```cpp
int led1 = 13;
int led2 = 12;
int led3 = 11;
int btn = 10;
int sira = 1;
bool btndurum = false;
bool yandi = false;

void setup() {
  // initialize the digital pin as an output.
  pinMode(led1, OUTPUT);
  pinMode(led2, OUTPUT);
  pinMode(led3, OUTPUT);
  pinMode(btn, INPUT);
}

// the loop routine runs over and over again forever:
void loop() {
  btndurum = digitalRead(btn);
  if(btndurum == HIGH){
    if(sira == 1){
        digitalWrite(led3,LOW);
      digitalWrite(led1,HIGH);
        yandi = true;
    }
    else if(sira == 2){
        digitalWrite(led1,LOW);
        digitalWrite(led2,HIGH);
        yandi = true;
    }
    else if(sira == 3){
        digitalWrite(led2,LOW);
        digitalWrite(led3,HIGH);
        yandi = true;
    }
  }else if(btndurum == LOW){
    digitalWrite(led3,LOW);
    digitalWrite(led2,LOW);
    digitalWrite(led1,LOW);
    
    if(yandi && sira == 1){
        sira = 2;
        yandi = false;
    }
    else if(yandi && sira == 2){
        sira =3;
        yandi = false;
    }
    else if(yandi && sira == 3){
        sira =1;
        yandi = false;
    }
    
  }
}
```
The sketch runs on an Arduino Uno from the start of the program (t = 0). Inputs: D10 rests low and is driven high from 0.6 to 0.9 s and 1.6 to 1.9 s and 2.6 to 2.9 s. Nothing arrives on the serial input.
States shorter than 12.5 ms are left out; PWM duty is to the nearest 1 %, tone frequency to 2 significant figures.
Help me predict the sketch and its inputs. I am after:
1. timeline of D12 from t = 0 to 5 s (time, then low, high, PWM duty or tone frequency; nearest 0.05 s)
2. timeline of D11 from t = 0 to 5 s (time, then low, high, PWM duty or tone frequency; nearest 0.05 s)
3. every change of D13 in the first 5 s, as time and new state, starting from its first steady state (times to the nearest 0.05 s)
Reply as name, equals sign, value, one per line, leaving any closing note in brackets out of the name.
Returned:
timeline of D12 from t = 0 to 5 s = 0 s low; 1.6 s high; 1.9 s low
timeline of D11 from t = 0 to 5 s = 0 s low; 2.6 s high; 2.9 s low
every change of D13 in the first 5 s, as time and new state, starting from its first steady state = 0 s low; 0.6 s high; 0.9 s low
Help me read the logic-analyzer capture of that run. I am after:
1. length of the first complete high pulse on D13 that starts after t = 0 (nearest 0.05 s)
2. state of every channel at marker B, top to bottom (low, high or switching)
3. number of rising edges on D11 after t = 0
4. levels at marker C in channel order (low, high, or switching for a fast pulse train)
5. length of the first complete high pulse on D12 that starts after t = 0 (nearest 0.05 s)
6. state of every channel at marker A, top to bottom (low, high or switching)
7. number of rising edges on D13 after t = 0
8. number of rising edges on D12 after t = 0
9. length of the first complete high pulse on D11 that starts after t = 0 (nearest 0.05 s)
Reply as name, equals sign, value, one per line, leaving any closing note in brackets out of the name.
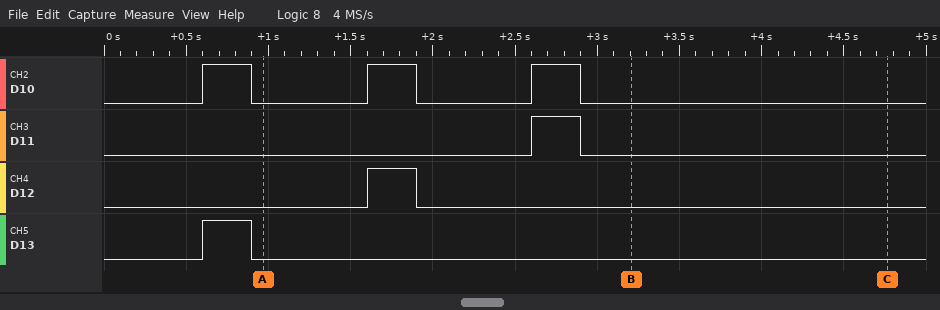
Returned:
length of the first complete high pulse on D13 that starts after t = 0 = 0.30 s
state of every channel at marker B, top to bottom = D10 low, D11 low, D12 low, D13 low
number of rising edges on D11 after t = 0 = 1
levels at marker C in channel order = D10 low, D11 low, D12 low, D13 low
length of the first complete high pulse on D12 that starts after t = 0 = 0.30 s
state of every channel at marker A, top to bottom = D10 low, D11 low, D12 low, D13 low
number of rising edges on D13 after t = 0 = 1
number of rising edges on D12 after t = 0 = 1
length of the first complete high pulse on D11 that starts after t = 0 = 0.30 s
